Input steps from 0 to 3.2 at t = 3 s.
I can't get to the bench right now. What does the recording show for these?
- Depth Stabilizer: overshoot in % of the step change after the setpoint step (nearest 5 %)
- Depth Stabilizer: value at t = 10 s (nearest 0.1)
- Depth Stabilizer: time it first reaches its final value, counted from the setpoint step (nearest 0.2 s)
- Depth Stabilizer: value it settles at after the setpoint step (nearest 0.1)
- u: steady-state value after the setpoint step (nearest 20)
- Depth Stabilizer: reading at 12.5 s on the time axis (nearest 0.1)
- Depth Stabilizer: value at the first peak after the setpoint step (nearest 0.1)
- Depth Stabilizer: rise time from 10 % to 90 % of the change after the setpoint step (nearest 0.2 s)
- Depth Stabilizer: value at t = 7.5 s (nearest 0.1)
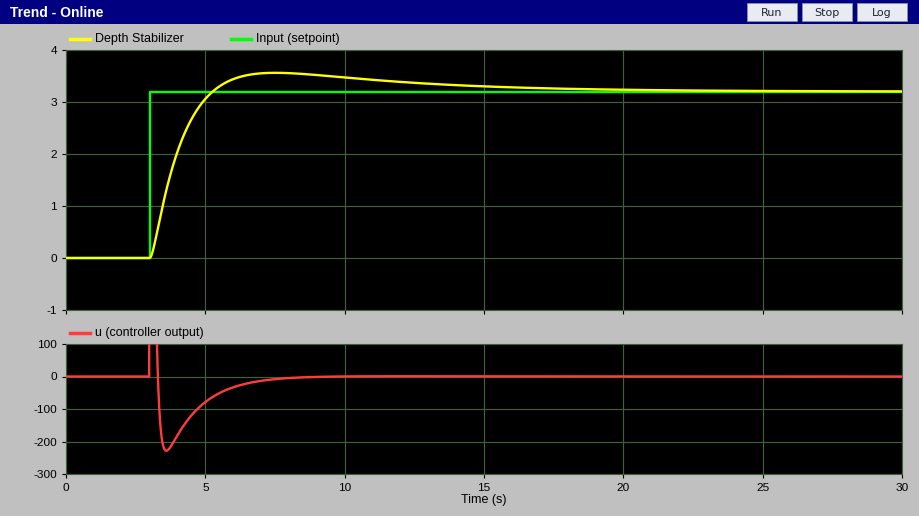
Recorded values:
10 %
3.5
2.2 s
3.2
0
3.4
3.6
1.6 s
3.6
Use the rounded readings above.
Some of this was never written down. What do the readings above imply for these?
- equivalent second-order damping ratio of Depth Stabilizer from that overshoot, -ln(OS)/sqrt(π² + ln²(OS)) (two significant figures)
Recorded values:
0.59
